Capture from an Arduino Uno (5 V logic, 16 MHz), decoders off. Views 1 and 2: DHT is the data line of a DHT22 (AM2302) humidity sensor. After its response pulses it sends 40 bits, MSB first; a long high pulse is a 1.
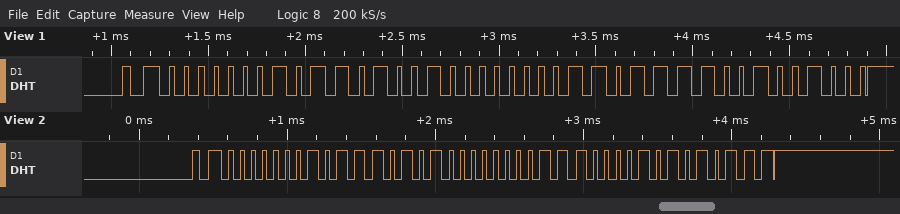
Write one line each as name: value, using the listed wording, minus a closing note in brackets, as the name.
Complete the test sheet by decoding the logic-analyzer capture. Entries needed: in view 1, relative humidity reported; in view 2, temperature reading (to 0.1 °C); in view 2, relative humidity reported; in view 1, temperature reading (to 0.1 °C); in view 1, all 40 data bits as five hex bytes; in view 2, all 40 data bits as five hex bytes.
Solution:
in view 1, relative humidity reported: 36.1 %
in view 2, temperature reading: 22.5 °C
in view 2, relative humidity reported: 37.3 %
in view 1, temperature reading: 22.2 °C
in view 1, all 40 data bits as five hex bytes: 01 69 00 DE 48
in view 2, all 40 data bits as five hex bytes: 01 75 00 E1 57
